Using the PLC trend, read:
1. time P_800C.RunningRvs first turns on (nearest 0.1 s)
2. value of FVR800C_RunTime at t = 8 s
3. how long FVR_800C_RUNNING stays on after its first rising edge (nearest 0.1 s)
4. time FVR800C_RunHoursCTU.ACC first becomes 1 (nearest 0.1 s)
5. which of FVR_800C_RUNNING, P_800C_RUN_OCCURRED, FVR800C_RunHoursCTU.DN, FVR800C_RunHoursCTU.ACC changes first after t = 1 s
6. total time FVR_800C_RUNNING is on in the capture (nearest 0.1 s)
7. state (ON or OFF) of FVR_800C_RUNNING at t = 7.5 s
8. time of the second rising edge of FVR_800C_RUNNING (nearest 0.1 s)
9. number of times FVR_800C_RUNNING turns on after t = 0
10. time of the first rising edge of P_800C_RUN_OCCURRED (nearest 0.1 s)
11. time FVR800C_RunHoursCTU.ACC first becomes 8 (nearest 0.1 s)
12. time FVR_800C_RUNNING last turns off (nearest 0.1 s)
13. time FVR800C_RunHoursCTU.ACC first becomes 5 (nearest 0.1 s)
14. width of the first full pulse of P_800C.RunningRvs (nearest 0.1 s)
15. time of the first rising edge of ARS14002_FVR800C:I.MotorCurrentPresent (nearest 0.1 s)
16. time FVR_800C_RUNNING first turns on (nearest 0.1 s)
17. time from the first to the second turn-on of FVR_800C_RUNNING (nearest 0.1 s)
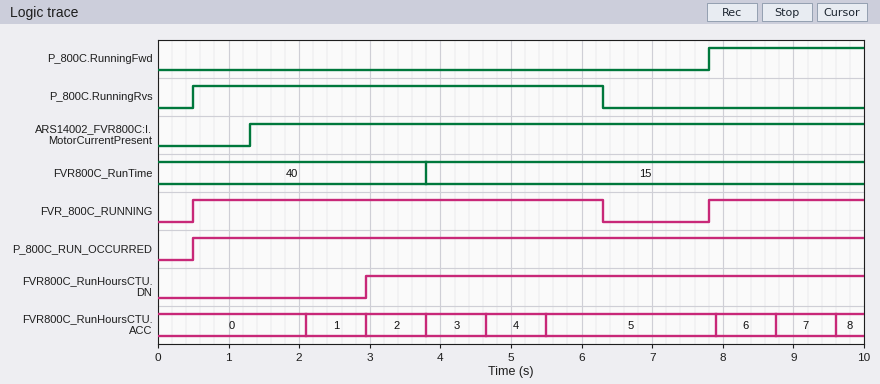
0.5 s
15
5.8 s
2.1 s
FVR800C_RunHoursCTU.ACC
8.0 s
OFF
7.8 s
2
0.5 s
9.6 s
6.3 s
5.5 s
5.8 s
1.3 s
0.5 s
7.3 s
